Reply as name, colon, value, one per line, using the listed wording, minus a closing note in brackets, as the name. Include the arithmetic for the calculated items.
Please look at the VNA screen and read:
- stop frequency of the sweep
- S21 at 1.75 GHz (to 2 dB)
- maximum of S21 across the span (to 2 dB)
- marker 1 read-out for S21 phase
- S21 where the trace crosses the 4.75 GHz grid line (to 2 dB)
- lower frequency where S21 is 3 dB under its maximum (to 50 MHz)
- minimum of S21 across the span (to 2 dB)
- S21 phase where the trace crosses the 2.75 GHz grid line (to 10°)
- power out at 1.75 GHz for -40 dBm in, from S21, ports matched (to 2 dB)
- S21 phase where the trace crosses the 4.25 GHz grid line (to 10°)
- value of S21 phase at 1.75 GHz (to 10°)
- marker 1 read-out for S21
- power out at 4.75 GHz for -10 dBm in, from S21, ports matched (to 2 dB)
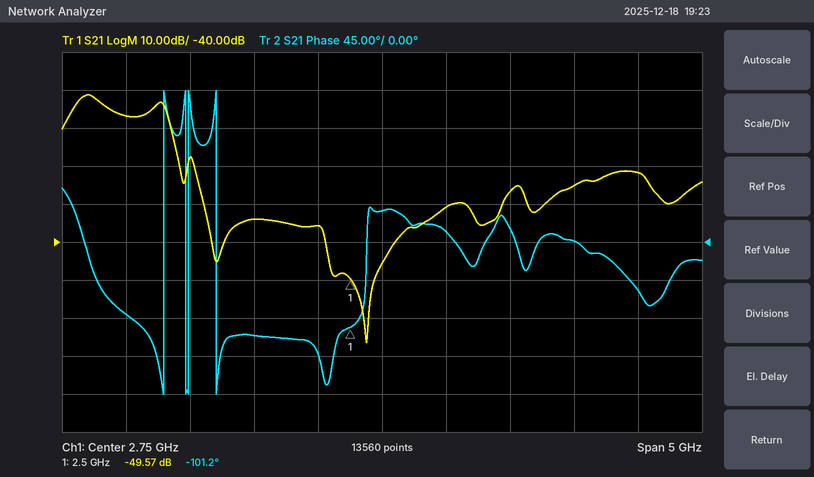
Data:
stop frequency of the sweep: 5.25 GHz
S21 at 1.75 GHz: -34 dB
maximum of S21 across the span: -2 dB
marker 1 read-out for S21 phase: -101.2°
S21 where the trace crosses the 4.75 GHz grid line: -22 dB
lower frequency where S21 is 3 dB under its maximum: 350 MHz
minimum of S21 across the span: -66 dB
S21 phase where the trace crosses the 2.75 GHz grid line: 40°
power out at 1.75 GHz for -40 dBm in, from S21, ports matched: -40 dBm + (-34 dB) = -74 dBm
S21 phase where the trace crosses the 4.25 GHz grid line: 0°
value of S21 phase at 1.75 GHz: -110°
marker 1 read-out for S21: -49.57 dB
power out at 4.75 GHz for -10 dBm in, from S21, ports matched: -10 dBm + (-22 dB) = -32 dBm
